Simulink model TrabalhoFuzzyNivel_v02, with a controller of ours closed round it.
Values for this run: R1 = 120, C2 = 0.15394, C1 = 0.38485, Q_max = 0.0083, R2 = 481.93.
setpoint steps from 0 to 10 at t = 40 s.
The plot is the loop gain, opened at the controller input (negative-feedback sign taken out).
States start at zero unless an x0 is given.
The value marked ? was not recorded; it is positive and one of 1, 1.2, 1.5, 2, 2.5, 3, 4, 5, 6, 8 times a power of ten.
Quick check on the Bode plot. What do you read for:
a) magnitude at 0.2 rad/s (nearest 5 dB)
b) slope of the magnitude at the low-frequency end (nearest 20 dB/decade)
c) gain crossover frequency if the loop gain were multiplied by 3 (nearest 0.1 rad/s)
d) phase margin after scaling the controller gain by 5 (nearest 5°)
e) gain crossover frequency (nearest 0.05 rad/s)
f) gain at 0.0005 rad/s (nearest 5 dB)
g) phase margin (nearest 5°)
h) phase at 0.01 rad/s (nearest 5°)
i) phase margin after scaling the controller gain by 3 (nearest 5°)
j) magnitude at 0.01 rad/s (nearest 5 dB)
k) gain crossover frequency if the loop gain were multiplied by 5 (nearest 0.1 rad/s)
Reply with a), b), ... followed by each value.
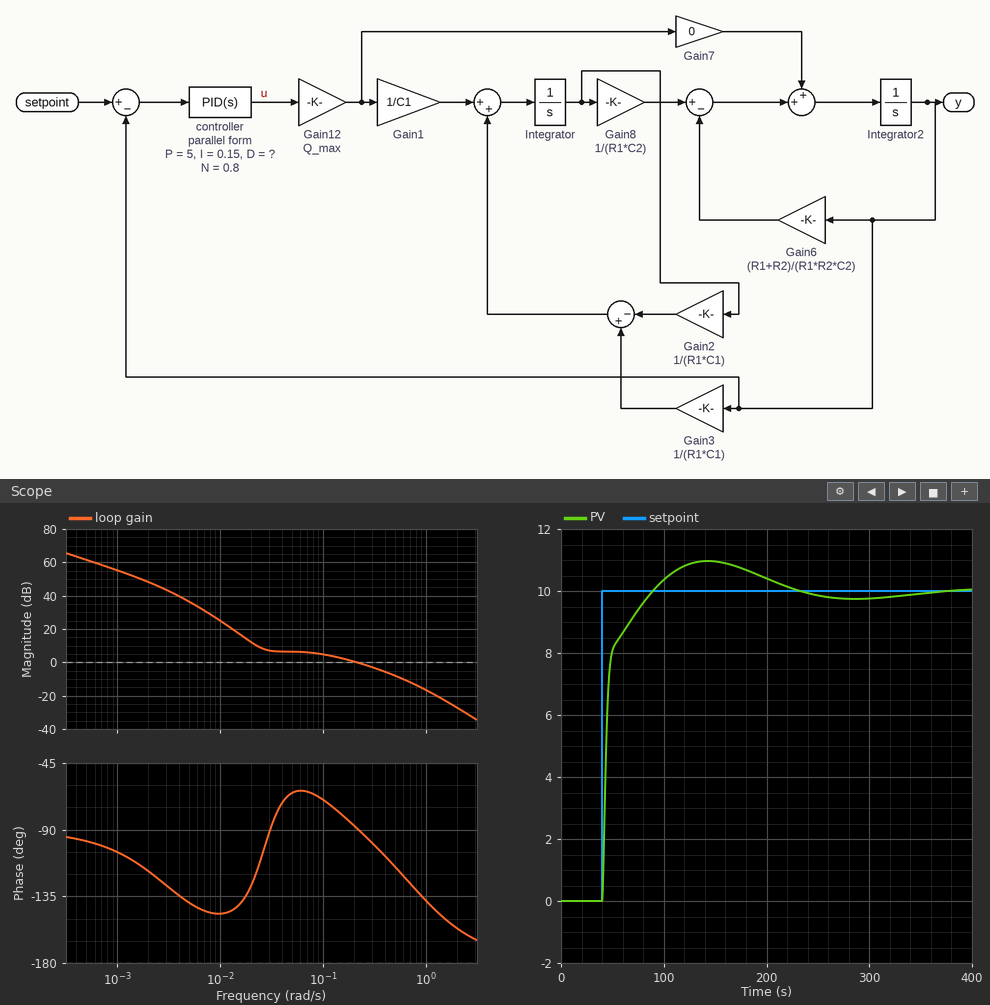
a) 0 dB
b) -20 dB/decade
c) 0.6 rad/s
d) 50°
e) 0.20 rad/s
f) 60 dB
g) 90°
h) -145°
i) 60°
j) 25 dB
k) 0.8 rad/s
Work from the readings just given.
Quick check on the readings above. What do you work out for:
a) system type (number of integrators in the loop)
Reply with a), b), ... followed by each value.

a) 1
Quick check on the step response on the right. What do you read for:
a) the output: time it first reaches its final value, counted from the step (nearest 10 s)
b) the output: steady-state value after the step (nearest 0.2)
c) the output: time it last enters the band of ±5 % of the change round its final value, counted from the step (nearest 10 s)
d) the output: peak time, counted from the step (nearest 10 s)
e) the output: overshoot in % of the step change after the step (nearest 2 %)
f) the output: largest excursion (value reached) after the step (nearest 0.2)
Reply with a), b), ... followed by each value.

a) 50 s
b) 10.0
c) 150 s
d) 100 s
e) 10 %
f) 11.0
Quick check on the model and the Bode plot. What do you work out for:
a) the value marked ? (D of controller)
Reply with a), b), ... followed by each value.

a) 200
